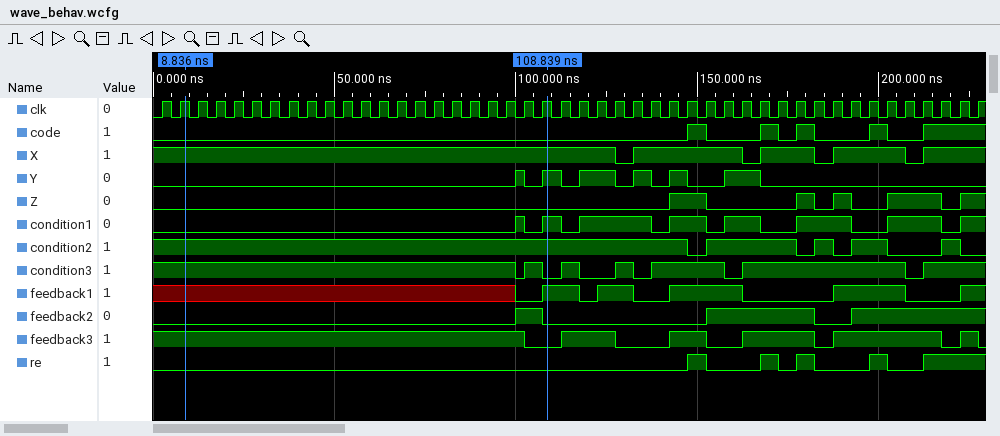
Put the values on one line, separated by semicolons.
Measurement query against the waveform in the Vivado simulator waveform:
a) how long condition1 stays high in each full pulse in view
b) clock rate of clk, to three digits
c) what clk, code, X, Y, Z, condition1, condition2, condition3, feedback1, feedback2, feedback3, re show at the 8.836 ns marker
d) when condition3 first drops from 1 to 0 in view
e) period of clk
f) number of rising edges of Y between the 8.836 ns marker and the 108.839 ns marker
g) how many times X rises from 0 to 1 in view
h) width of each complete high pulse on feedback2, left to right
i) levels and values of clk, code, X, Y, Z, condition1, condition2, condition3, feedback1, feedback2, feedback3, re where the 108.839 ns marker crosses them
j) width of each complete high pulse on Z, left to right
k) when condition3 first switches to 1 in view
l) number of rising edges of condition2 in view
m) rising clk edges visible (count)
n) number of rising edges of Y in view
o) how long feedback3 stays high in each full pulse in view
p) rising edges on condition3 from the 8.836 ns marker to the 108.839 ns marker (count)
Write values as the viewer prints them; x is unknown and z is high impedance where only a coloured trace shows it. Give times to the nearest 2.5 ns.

2.5 ns, 5 ns, 20 ns, 10 ns, 10 ns, 15 ns, 15 ns; 200 MHz; clk=1, code=0, X=1, Y=0, Z=0, condition1=0, condition2=1, condition3=1, feedback1=x, feedback2=0, feedback3=1, re=0; 100 ns; 5 ns; 2; 4; 7.5 ns, 30 ns; clk=1, code=0, X=1, Y=1, Z=0, condition1=1, condition2=1, condition3=0, feedback1=1, feedback2=0, feedback3=0, re=0; 10 ns, 5 ns, 5 ns, 15 ns; 102.5 ns; 4; 46; 6; 15 ns, 10 ns, 20 ns, 30 ns, 5 ns; 1
